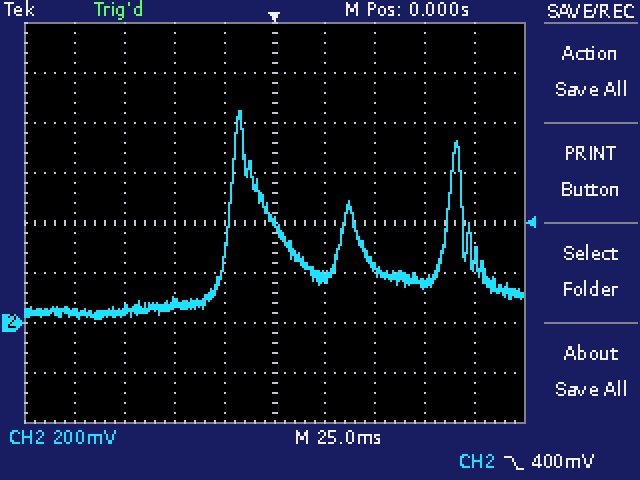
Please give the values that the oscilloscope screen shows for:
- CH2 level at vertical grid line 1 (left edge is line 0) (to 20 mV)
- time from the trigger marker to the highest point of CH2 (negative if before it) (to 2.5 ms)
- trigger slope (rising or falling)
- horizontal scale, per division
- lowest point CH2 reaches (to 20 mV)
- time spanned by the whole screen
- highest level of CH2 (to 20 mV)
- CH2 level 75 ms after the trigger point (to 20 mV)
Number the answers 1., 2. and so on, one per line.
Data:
1. 40 mV
2. -17.5 ms
3. falling
4. 25 ms
5. 20 mV
6. 250 ms
7. 840 mV
8. 160 mV
